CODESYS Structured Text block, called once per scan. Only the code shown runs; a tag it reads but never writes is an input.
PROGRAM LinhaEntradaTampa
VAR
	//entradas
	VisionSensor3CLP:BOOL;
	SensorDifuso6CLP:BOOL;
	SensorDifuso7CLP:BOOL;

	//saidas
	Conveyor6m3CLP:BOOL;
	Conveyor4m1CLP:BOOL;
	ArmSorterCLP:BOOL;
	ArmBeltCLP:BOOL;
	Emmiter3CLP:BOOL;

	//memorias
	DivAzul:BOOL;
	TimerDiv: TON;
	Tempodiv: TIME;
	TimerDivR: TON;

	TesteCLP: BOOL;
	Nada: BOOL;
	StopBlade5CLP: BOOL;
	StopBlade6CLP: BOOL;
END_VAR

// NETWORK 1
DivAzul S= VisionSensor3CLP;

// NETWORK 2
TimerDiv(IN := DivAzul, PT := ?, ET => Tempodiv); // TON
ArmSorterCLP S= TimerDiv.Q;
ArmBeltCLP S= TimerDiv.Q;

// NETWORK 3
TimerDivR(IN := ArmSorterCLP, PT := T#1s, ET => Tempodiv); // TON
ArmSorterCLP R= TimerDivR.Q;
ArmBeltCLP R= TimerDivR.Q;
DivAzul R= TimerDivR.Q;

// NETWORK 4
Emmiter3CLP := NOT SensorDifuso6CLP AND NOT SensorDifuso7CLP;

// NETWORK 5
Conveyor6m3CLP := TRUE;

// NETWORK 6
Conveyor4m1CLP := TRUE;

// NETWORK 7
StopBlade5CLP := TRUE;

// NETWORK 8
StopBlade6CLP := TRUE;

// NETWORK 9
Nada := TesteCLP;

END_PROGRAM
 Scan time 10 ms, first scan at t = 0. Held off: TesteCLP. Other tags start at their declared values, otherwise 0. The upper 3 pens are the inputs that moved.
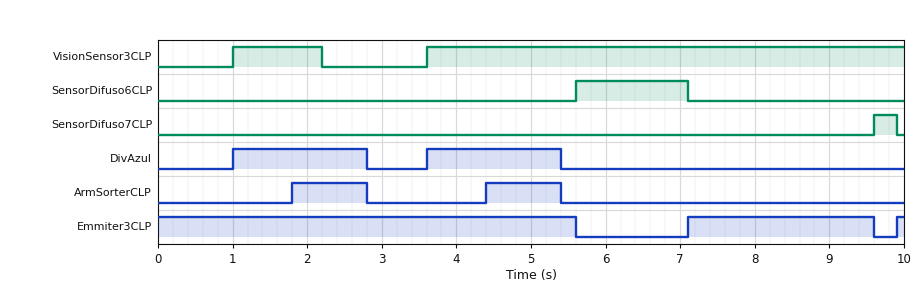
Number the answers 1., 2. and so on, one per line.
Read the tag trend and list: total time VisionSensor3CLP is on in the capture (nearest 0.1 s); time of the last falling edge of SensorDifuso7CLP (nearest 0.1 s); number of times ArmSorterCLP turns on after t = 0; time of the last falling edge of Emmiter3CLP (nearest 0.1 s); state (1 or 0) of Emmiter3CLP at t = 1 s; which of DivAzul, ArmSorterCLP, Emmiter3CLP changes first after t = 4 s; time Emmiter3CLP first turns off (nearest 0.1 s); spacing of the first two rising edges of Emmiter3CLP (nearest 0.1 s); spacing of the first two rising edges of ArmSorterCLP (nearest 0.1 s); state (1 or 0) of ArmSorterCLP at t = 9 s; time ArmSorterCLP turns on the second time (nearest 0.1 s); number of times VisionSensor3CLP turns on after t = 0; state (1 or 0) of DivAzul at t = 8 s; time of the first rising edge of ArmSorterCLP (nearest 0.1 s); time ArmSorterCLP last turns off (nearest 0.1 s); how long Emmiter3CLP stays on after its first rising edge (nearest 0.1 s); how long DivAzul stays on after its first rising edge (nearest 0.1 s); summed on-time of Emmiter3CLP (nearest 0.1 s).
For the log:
1. 7.6 s
2. 9.9 s
3. 2
4. 9.6 s
5. 1
6. ArmSorterCLP
7. 5.6 s
8. 2.8 s
9. 2.6 s
10. 0
11. 4.4 s
12. 2
13. 0
14. 1.8 s
15. 5.4 s
16. 2.5 s
17. 1.8 s
18. 8.2 s
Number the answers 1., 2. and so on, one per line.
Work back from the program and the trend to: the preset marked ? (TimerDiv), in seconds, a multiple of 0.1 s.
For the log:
1. 0.8 s
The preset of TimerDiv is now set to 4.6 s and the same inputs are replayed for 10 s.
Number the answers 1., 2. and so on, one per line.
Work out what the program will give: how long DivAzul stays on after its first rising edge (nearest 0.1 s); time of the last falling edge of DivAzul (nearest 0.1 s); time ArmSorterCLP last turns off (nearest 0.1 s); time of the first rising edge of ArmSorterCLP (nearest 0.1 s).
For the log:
1. 5.6 s
2. 6.6 s
3. 6.6 s
4. 5.6 s
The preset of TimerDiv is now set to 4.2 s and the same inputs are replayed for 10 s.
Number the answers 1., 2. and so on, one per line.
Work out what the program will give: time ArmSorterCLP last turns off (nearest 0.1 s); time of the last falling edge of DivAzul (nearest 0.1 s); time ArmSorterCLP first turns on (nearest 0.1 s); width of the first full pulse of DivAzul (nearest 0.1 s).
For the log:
1. 6.2 s
2. 6.2 s
3. 5.2 s
4. 5.2 s
